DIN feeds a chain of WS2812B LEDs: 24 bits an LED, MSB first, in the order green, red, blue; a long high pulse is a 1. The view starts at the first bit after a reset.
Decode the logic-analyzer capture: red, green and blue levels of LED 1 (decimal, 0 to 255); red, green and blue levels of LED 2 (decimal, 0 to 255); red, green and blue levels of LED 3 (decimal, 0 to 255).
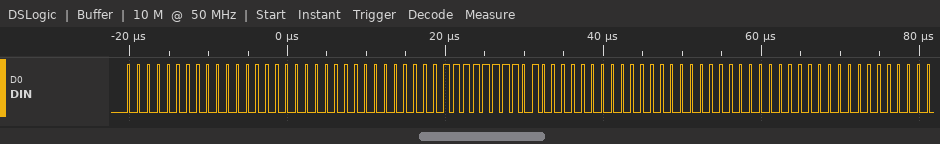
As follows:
0, 0, 0
255, 0, 64
0, 0, 0
